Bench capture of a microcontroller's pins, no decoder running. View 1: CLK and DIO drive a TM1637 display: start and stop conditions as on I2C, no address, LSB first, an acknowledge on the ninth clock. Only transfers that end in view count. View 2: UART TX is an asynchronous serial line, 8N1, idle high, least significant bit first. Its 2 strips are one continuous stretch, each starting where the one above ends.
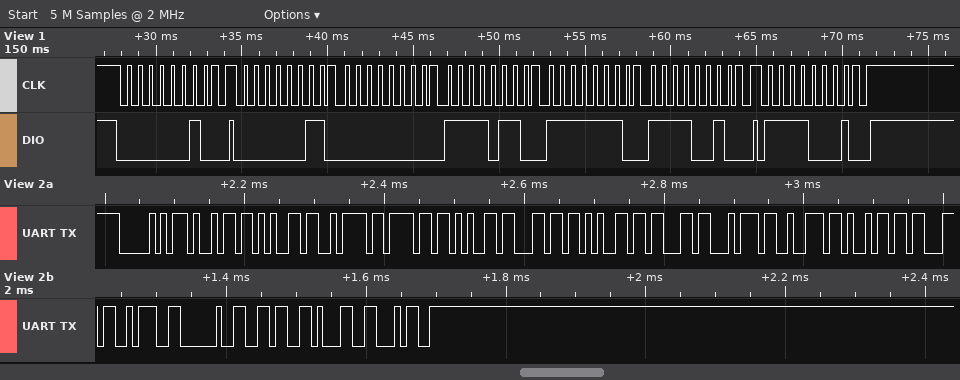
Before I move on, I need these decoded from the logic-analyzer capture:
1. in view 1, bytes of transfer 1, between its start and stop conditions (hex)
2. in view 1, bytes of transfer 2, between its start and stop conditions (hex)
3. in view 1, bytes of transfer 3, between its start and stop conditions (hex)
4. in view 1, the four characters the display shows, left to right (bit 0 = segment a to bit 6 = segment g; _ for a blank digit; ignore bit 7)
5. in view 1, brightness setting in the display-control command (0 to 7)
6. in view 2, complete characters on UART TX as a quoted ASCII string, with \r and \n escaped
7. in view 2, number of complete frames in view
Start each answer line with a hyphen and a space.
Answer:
- 40
- C0 00 6F 7F 4F
- 8F
- _983
- 7
- "Piezoelectric: 614"
- 18
